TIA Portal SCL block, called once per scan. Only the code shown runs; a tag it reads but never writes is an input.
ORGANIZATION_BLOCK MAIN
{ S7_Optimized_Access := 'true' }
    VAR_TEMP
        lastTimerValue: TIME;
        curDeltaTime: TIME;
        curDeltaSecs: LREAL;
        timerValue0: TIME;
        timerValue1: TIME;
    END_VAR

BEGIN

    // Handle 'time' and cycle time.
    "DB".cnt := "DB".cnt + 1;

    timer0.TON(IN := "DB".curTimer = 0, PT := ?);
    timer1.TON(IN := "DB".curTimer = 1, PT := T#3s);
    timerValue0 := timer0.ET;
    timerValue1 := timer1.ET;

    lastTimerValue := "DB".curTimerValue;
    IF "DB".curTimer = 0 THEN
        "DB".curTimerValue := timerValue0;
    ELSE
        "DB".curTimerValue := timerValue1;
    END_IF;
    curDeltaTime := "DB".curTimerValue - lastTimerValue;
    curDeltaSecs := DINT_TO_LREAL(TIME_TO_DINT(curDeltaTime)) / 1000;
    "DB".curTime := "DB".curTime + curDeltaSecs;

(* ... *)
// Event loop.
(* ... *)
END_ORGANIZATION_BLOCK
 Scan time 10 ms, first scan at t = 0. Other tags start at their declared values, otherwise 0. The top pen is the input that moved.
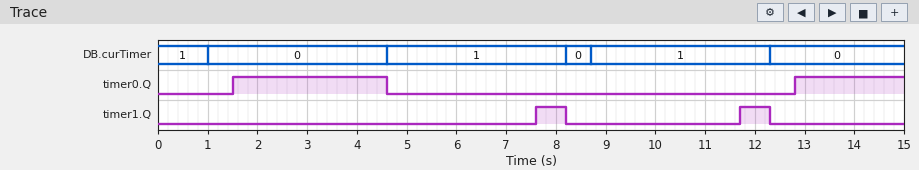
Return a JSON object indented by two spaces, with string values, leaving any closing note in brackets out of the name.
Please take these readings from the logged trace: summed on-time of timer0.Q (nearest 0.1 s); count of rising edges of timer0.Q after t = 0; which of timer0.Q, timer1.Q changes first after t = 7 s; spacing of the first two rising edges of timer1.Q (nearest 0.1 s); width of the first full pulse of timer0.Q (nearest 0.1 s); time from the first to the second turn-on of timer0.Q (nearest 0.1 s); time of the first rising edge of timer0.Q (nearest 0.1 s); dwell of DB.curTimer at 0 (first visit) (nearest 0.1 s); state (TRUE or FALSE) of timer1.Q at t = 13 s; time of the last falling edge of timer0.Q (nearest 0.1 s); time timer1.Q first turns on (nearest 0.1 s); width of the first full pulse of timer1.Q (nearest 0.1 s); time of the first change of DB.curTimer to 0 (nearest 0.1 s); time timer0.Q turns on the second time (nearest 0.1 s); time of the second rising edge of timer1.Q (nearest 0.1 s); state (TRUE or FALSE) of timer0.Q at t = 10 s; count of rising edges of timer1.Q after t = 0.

{
  "summed on-time of timer0.Q": "5.3 s",
  "count of rising edges of timer0.Q after t = 0": "2",
  "which of timer0.Q, timer1.Q changes first after t = 7 s": "timer1.Q",
  "spacing of the first two rising edges of timer1.Q": "4.1 s",
  "width of the first full pulse of timer0.Q": "3.1 s",
  "time from the first to the second turn-on of timer0.Q": "11.3 s",
  "time of the first rising edge of timer0.Q": "1.5 s",
  "dwell of DB.curTimer at 0 (first visit)": "3.6 s",
  "state (TRUE or FALSE) of timer1.Q at t = 13 s": "FALSE",
  "time of the last falling edge of timer0.Q": "4.6 s",
  "time timer1.Q first turns on": "7.6 s",
  "width of the first full pulse of timer1.Q": "0.6 s",
  "time of the first change of DB.curTimer to 0": "1.0 s",
  "time timer0.Q turns on the second time": "12.8 s",
  "time of the second rising edge of timer1.Q": "11.7 s",
  "state (TRUE or FALSE) of timer0.Q at t = 10 s": "FALSE",
  "count of rising edges of timer1.Q after t = 0": "2"
}
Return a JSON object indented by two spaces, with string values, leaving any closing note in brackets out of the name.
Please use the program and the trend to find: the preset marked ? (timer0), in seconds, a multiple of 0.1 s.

{
  "the preset marked ? (timer0), in seconds, a multiple of 0.1 s": "0.5 s"
}
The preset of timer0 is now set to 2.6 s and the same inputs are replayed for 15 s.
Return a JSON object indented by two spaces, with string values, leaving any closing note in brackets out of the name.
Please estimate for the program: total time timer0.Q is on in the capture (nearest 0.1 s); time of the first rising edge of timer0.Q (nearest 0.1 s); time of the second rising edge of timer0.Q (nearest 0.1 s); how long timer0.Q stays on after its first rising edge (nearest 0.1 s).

{
  "total time timer0.Q is on in the capture": "1.1 s",
  "time of the first rising edge of timer0.Q": "3.6 s",
  "time of the second rising edge of timer0.Q": "14.9 s",
  "how long timer0.Q stays on after its first rising edge": "1.0 s"
}
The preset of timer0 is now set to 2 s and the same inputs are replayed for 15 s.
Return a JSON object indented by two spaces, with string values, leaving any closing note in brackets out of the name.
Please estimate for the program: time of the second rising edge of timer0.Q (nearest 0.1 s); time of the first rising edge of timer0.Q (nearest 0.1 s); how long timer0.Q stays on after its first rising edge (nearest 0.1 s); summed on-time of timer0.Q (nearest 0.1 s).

{
  "time of the second rising edge of timer0.Q": "14.3 s",
  "time of the first rising edge of timer0.Q": "3.0 s",
  "how long timer0.Q stays on after its first rising edge": "1.6 s",
  "summed on-time of timer0.Q": "2.3 s"
}
